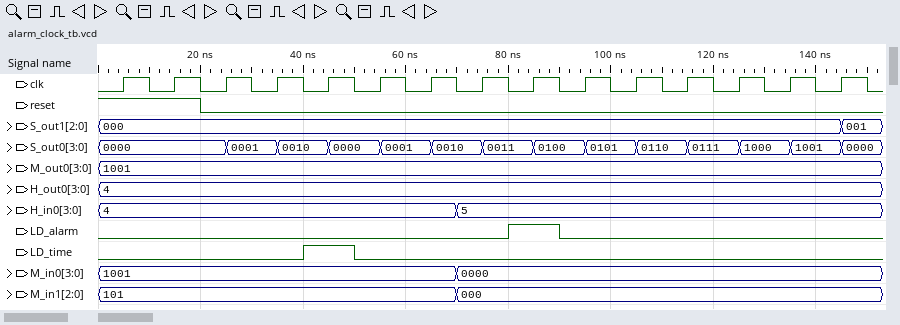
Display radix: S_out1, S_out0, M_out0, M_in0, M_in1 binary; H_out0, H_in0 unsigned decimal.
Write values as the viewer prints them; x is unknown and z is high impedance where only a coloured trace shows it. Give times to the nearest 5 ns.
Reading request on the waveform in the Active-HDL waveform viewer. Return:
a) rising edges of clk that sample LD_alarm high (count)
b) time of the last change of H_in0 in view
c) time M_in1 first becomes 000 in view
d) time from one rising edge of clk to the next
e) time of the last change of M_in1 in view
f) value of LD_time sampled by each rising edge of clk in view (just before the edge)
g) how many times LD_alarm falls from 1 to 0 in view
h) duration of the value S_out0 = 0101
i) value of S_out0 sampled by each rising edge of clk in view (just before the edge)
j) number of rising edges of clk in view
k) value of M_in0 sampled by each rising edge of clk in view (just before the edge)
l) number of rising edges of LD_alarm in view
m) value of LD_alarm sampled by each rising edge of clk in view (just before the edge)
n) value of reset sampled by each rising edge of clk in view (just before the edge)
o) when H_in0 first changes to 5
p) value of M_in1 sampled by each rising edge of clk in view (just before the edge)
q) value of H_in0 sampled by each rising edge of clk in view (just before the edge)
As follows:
1
70 ns
70 ns
10 ns
70 ns
0 0 0 0 1 0 0 0 0 0 0 0 0 0 0
1
10 ns
0000, 0000, 0000, 0001, 0010, 0000, 0001, 0010, 0011, 0100, 0101, 0110, 0111, 1000, 1001
15
1001, 1001, 1001, 1001, 1001, 1001, 1001, 0000, 0000, 0000, 0000, 0000, 0000, 0000, 0000
1
0 0 0 0 0 0 0 0 1 0 0 0 0 0 0
1 1 0 0 0 0 0 0 0 0 0 0 0 0 0
70 ns
101, 101, 101, 101, 101, 101, 101, 000, 000, 000, 000, 000, 000, 000, 000
4, 4, 4, 4, 4, 4, 4, 5, 5, 5, 5, 5, 5, 5, 5
